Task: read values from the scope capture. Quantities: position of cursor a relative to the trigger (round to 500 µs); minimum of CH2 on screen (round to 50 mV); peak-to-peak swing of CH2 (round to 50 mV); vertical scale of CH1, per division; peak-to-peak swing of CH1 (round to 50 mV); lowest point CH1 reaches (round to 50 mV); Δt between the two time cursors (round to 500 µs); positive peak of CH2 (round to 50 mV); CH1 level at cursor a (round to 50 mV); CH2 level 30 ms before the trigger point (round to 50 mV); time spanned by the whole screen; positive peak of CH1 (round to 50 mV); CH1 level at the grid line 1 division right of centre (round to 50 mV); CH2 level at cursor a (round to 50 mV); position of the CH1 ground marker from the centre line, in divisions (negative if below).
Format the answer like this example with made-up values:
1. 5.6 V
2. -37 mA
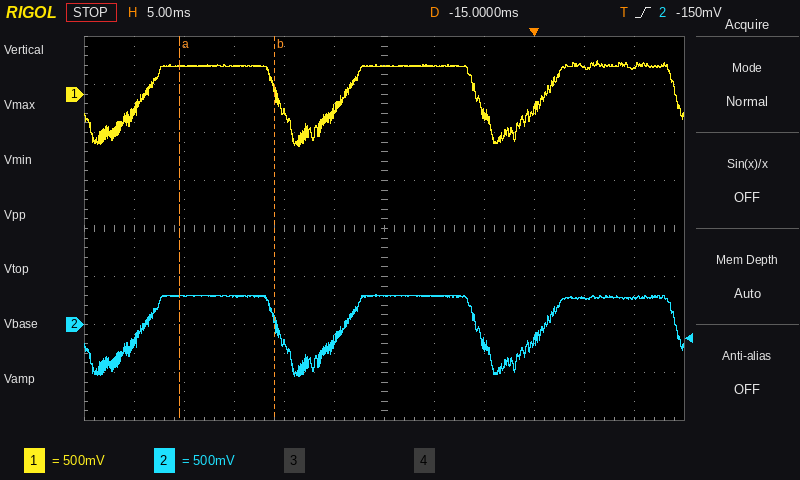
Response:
1. -35.5 ms
2. -550 mV
3. 850 mV
4. 500 mV
5. 900 mV
6. -550 mV
7. 9.5 ms
8. 300 mV
9. 300 mV
10. 300 mV
11. 60 ms
12. 350 mV
13. 300 mV
14. 300 mV
15. +2.8 div
